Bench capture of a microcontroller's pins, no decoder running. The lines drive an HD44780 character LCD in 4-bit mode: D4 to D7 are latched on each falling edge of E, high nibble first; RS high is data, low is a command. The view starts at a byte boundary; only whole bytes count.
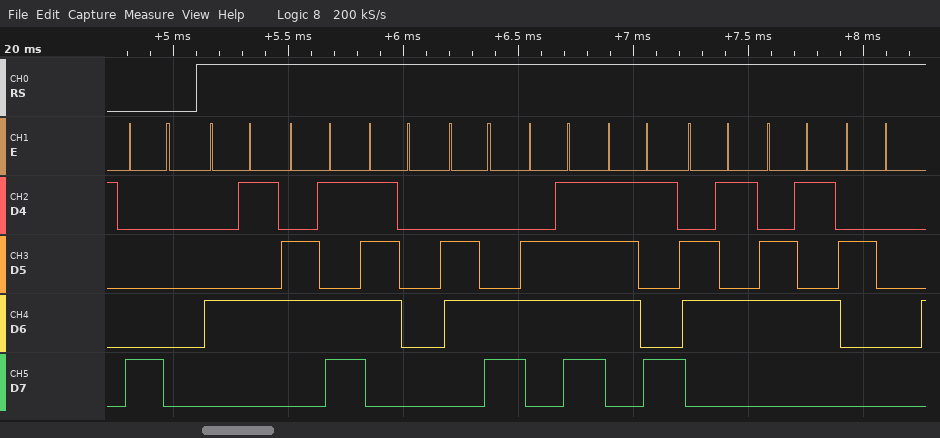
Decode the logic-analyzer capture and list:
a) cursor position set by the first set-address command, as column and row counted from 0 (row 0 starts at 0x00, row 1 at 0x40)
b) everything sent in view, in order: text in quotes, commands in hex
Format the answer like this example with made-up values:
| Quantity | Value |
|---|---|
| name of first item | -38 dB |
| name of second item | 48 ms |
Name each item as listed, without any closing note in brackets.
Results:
| Quantity | Value |
|---|---|
| cursor position set by the first set-address command, as column and row counted from 0 | column 0, row 0 |
| everything sent in view, in order: text in quotes, commands in hex | 0x80 "Employee " |
